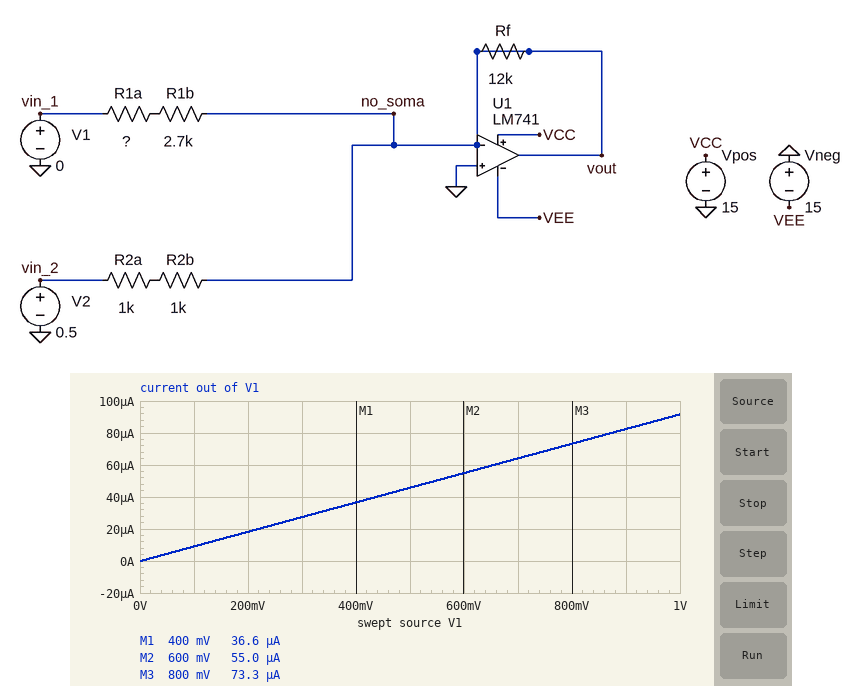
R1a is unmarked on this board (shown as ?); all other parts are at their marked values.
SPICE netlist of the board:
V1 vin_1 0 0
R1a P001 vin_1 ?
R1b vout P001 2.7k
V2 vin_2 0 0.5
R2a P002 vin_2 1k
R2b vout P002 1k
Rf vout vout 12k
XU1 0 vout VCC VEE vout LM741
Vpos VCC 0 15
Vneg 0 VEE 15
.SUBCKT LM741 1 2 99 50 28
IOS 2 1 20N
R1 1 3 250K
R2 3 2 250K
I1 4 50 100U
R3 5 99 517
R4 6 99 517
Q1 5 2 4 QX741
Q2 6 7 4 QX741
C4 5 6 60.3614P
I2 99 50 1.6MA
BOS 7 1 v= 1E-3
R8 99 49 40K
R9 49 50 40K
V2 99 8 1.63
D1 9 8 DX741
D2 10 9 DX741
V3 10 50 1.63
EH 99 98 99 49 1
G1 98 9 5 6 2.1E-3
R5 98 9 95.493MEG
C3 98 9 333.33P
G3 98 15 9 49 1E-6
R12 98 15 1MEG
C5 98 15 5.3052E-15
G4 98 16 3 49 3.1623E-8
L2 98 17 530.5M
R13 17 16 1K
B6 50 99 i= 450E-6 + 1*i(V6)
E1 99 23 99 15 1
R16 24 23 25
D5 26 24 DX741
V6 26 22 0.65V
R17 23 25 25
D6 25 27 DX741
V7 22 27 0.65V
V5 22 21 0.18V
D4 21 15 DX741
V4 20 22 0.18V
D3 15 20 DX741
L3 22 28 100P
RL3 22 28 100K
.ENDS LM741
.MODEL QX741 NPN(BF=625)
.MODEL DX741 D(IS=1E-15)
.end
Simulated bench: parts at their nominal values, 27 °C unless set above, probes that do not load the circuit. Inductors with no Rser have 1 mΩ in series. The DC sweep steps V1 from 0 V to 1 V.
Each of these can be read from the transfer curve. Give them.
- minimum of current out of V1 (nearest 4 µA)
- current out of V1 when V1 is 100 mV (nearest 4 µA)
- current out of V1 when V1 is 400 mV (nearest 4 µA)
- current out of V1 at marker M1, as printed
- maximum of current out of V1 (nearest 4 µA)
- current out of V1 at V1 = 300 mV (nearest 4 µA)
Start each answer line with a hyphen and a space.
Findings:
- 0 A
- 8 µA
- 36 µA
- 36.6 µA
- 92 µA
- 28 µA
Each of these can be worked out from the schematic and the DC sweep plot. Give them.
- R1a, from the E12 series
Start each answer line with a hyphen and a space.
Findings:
- 8.2 kΩ
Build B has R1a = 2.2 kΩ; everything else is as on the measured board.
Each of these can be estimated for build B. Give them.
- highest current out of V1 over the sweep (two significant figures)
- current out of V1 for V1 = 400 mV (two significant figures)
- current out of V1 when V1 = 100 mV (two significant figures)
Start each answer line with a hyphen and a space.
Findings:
- 200 µA
- 81 µA
- 20 µA
